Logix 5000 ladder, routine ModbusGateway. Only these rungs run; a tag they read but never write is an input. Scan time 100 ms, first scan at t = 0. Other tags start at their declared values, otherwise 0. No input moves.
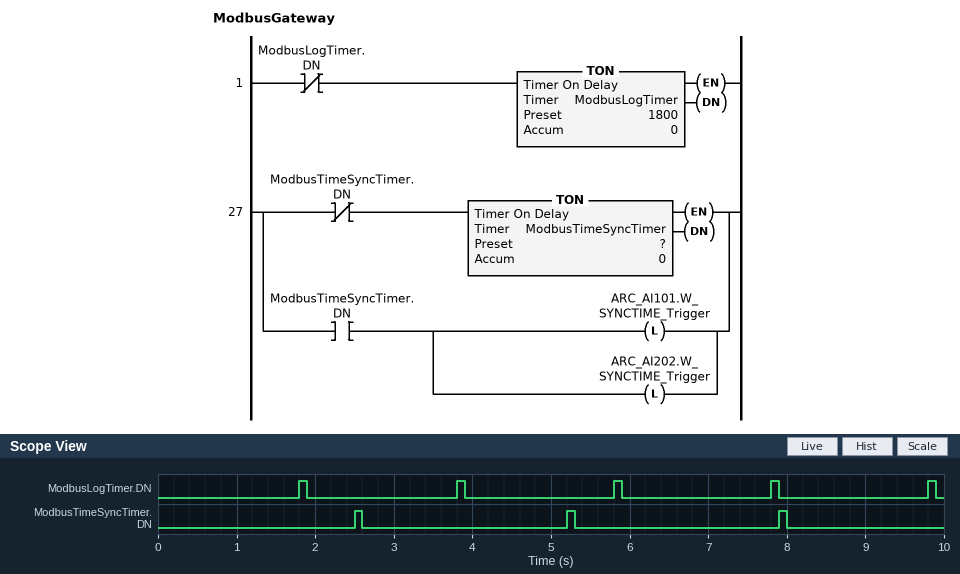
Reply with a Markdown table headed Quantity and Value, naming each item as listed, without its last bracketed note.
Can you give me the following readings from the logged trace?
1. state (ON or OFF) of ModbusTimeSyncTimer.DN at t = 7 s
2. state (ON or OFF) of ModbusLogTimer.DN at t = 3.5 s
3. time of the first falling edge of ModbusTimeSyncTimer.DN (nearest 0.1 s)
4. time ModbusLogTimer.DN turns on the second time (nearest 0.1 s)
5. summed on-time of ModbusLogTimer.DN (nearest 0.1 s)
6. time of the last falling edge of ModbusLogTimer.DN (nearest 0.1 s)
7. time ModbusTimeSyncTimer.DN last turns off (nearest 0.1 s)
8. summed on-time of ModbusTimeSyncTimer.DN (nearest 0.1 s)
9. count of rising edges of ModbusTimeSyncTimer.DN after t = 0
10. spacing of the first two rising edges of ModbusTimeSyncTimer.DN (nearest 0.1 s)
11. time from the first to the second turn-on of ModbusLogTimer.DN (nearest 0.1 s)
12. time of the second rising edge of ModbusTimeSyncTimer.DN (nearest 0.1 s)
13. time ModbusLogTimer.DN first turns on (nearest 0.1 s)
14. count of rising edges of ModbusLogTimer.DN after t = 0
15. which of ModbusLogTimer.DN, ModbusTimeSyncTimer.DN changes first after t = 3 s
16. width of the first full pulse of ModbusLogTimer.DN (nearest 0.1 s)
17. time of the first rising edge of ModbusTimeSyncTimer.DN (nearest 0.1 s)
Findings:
| Quantity | Value |
|---|---|
| state (ON or OFF) of ModbusTimeSyncTimer.DN at t = 7 s | OFF |
| state (ON or OFF) of ModbusLogTimer.DN at t = 3.5 s | OFF |
| time of the first falling edge of ModbusTimeSyncTimer.DN | 2.6 s |
| time ModbusLogTimer.DN turns on the second time | 3.8 s |
| summed on-time of ModbusLogTimer.DN | 0.5 s |
| time of the last falling edge of ModbusLogTimer.DN | 9.9 s |
| time ModbusTimeSyncTimer.DN last turns off | 8.0 s |
| summed on-time of ModbusTimeSyncTimer.DN | 0.3 s |
| count of rising edges of ModbusTimeSyncTimer.DN after t = 0 | 3 |
| spacing of the first two rising edges of ModbusTimeSyncTimer.DN | 2.7 s |
| time from the first to the second turn-on of ModbusLogTimer.DN | 2.0 s |
| time of the second rising edge of ModbusTimeSyncTimer.DN | 5.2 s |
| time ModbusLogTimer.DN first turns on | 1.8 s |
| count of rising edges of ModbusLogTimer.DN after t = 0 | 5 |
| which of ModbusLogTimer.DN, ModbusTimeSyncTimer.DN changes first after t = 3 s | ModbusLogTimer.DN |
| width of the first full pulse of ModbusLogTimer.DN | 0.1 s |
| time of the first rising edge of ModbusTimeSyncTimer.DN | 2.5 s |
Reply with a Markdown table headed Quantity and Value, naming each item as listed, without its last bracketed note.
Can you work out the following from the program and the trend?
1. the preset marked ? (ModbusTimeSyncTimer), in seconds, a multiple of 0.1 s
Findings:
| Quantity | Value |
|---|---|
| the preset marked ? (ModbusTimeSyncTimer), in seconds, a multiple of 0.1 s | 2.5 s |
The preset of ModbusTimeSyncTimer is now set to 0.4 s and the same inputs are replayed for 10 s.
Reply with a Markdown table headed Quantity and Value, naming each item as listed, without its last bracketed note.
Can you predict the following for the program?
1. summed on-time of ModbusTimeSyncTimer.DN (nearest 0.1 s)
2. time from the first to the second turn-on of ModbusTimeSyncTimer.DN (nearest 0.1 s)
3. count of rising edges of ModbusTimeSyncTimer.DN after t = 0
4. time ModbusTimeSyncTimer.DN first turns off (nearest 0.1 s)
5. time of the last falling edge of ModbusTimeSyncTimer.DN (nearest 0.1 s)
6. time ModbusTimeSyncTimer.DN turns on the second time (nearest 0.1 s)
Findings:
| Quantity | Value |
|---|---|
| summed on-time of ModbusTimeSyncTimer.DN | 1.6 s |
| time from the first to the second turn-on of ModbusTimeSyncTimer.DN | 0.6 s |
| count of rising edges of ModbusTimeSyncTimer.DN after t = 0 | 16 |
| time ModbusTimeSyncTimer.DN first turns off | 0.5 s |
| time of the last falling edge of ModbusTimeSyncTimer.DN | 9.5 s |
| time ModbusTimeSyncTimer.DN turns on the second time | 1.0 s |
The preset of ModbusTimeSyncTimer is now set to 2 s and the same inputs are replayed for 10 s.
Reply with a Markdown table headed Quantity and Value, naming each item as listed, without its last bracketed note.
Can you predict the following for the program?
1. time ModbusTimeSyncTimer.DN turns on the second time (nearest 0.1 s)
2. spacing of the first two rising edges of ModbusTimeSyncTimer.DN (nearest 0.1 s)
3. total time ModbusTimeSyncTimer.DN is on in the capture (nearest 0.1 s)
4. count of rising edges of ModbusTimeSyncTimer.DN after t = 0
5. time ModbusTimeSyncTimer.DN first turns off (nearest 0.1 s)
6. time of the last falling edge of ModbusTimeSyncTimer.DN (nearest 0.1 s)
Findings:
| Quantity | Value |
|---|---|
| time ModbusTimeSyncTimer.DN turns on the second time | 4.2 s |
| spacing of the first two rising edges of ModbusTimeSyncTimer.DN | 2.2 s |
| total time ModbusTimeSyncTimer.DN is on in the capture | 0.4 s |
| count of rising edges of ModbusTimeSyncTimer.DN after t = 0 | 4 |
| time ModbusTimeSyncTimer.DN first turns off | 2.1 s |
| time of the last falling edge of ModbusTimeSyncTimer.DN | 8.7 s |
